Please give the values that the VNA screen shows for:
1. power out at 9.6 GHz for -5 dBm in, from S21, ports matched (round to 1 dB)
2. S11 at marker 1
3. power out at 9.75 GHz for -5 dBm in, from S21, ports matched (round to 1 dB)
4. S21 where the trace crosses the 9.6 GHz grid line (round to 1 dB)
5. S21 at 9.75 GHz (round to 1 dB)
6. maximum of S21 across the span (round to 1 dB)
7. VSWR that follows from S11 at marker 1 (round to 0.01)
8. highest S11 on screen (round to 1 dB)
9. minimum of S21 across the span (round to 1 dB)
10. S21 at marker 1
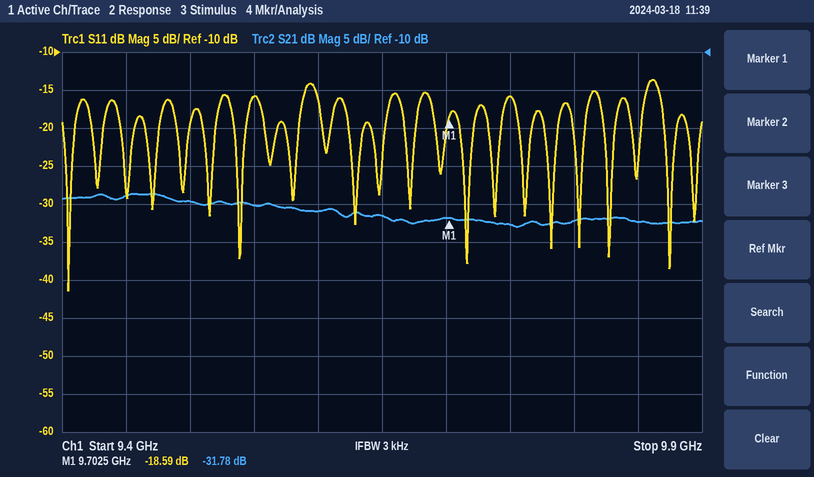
-36 dBm
-18.59 dB
-38 dBm
-31 dB
-33 dB
-29 dB
1.27
-14 dB
-33 dB
-31.78 dB
